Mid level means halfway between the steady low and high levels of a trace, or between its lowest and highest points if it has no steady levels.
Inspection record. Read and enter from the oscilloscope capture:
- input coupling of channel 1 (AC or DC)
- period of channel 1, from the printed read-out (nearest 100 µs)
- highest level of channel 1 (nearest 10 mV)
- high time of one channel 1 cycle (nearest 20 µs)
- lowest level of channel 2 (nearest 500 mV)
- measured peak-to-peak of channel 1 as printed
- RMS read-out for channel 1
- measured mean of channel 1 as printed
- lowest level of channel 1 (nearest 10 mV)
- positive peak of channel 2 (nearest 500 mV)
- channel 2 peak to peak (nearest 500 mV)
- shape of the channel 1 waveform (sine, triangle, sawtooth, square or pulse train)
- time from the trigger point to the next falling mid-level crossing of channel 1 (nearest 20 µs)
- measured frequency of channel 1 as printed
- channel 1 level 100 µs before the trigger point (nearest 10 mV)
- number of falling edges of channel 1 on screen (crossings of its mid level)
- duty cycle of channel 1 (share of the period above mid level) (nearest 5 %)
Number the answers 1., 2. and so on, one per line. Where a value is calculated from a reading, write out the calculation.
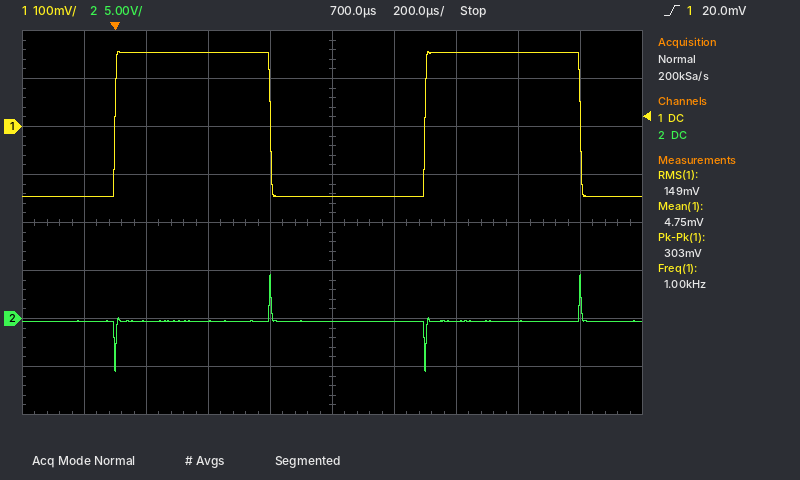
1. DC
2. 1 / 1.00 kHz ≈ 1.0 ms
3. 160 mV
4. 500 µs
5. -5.5 V
6. 303 mV
7. 149 mV
8. 4.75 mV
9. -150 mV
10. 4.5 V
11. 4.5 V − (-5.5 V) = 10.0 V
12. square
13. 500 µs
14. 1.00 kHz
15. -150 mV
16. 2
17. 50 %
